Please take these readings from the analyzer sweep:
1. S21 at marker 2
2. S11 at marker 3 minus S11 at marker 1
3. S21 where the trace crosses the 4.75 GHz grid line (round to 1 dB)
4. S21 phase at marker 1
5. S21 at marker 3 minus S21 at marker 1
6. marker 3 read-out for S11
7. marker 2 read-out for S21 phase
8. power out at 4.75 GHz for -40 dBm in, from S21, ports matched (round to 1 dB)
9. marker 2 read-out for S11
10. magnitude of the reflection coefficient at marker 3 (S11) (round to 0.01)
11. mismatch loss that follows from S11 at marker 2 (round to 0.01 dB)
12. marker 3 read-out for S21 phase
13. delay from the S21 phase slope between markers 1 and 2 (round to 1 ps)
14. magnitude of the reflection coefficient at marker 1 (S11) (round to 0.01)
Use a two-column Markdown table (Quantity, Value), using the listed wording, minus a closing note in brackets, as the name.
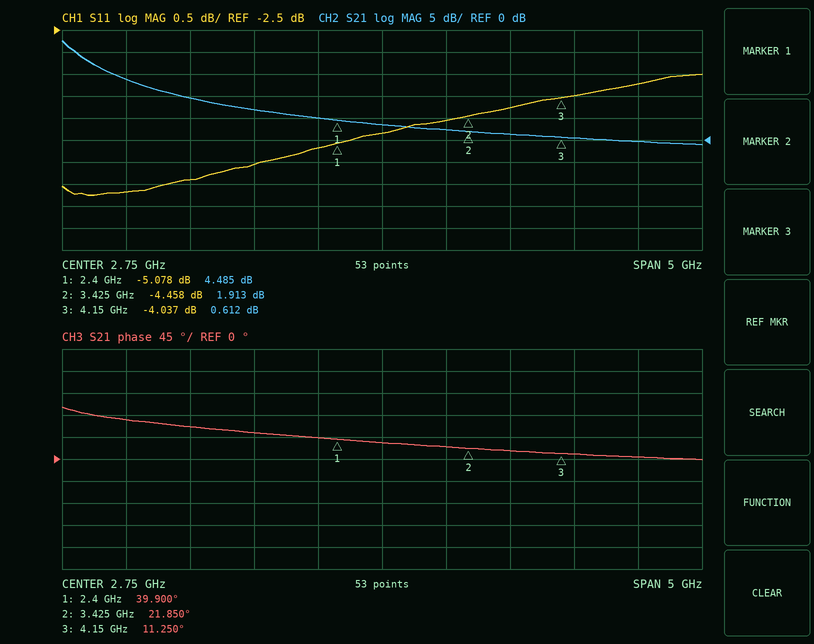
| Quantity | Value |
|---|---|
| S21 at marker 2 | 1.913 dB |
| S11 at marker 3 minus S11 at marker 1 | 1.041 dB |
| S21 where the trace crosses the 4.75 GHz grid line | 0 dB |
| S21 phase at marker 1 | 39.900° |
| S21 at marker 3 minus S21 at marker 1 | -3.873 dB |
| marker 3 read-out for S11 | -4.037 dB |
| marker 2 read-out for S21 phase | 21.850° |
| power out at 4.75 GHz for -40 dBm in, from S21, ports matched | -40 dBm |
| marker 2 read-out for S11 | -4.458 dB |
| magnitude of the reflection coefficient at marker 3 (S11) | 0.63 |
| mismatch loss that follows from S11 at marker 2 | 1.93 dB |
| marker 3 read-out for S21 phase | 11.250° |
| delay from the S21 phase slope between markers 1 and 2 | 49 ps |
| magnitude of the reflection coefficient at marker 1 (S11) | 0.56 |
